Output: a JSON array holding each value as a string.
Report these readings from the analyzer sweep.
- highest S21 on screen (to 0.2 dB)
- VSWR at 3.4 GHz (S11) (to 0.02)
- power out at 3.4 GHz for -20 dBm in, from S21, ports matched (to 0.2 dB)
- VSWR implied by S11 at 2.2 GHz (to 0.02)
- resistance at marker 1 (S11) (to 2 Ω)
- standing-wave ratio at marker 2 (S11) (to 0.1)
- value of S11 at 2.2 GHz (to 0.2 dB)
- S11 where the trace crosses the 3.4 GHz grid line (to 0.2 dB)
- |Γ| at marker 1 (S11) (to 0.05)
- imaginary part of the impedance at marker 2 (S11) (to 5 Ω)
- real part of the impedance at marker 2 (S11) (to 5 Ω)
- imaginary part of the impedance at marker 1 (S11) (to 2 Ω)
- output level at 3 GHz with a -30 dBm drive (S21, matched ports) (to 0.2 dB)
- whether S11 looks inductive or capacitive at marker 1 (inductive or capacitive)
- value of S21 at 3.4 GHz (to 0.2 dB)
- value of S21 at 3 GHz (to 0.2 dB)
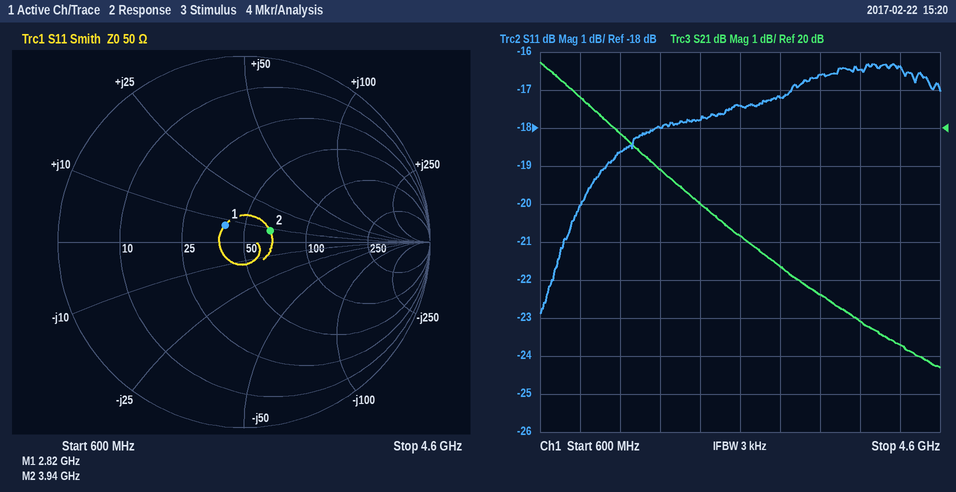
["21.8 dB", "1.34", "-4.4 dBm", "1.30", "40 Ω", "1.4", "-17.8 dB", "-16.6 dB", "0.15", "+10 Ω", "65 Ω", "+8 Ω", "-13.6 dBm", "inductive", "15.6 dB", "16.4 dB"]
